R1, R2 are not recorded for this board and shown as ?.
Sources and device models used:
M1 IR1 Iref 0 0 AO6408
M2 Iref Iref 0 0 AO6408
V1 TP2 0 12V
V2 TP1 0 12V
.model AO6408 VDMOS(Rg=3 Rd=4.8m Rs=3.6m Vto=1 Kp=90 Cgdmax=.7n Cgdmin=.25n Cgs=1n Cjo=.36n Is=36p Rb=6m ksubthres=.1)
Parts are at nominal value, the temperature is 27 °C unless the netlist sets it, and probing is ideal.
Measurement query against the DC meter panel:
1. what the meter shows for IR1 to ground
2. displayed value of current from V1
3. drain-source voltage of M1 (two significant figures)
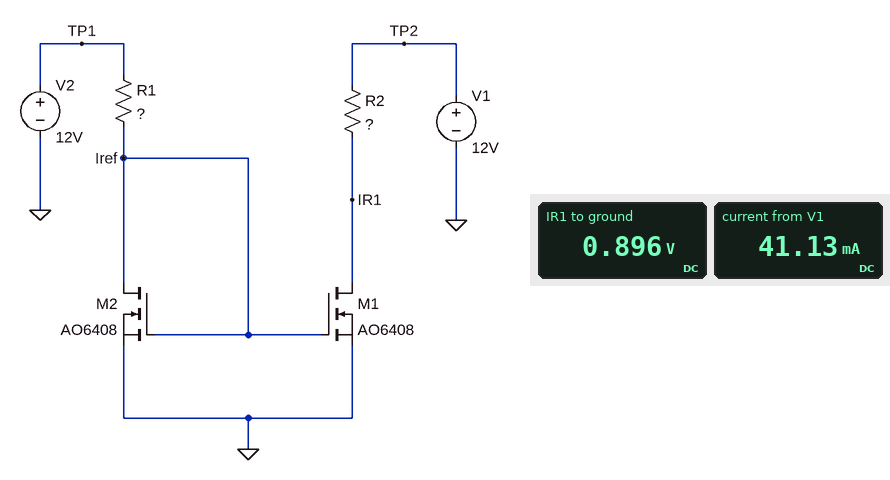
0.896 V
41.13 mA
900 mV
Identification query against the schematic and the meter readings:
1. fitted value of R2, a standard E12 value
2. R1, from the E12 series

270 Ω
270 Ω
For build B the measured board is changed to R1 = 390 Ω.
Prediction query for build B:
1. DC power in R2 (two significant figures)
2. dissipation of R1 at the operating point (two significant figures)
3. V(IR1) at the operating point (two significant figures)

220 mW
320 mW
4.3 V
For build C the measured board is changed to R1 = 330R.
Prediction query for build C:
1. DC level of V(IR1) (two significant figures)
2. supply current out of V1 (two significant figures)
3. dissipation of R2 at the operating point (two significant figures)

2.9 V
34 mA
310 mW
